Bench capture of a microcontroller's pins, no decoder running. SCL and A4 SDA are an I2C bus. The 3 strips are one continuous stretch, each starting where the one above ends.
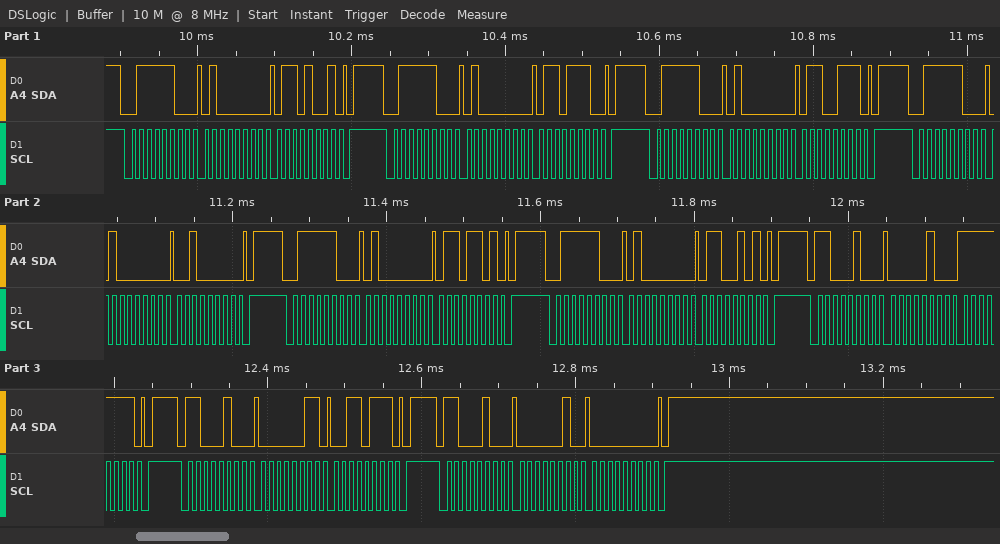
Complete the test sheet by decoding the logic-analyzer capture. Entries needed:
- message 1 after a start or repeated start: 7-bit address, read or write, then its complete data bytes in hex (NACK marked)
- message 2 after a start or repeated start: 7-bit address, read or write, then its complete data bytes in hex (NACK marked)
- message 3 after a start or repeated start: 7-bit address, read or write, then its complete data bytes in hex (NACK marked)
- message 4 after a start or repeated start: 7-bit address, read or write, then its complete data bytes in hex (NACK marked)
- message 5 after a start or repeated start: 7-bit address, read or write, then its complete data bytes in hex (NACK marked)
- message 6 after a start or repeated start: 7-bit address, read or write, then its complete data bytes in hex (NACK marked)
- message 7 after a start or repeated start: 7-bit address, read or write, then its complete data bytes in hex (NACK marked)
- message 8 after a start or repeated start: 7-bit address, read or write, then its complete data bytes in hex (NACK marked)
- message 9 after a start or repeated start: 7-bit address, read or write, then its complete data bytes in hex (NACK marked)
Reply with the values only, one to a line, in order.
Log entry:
0x3E write: 40 69
0x3E write: 40 6E
0x3E write: 40 67
0x3E write: 40 20
0x3E write: 40 6D
0x3E write: 40 65
0x62 write: 04 FF
0x62 write: 03 37
0x62 write: 02 00
